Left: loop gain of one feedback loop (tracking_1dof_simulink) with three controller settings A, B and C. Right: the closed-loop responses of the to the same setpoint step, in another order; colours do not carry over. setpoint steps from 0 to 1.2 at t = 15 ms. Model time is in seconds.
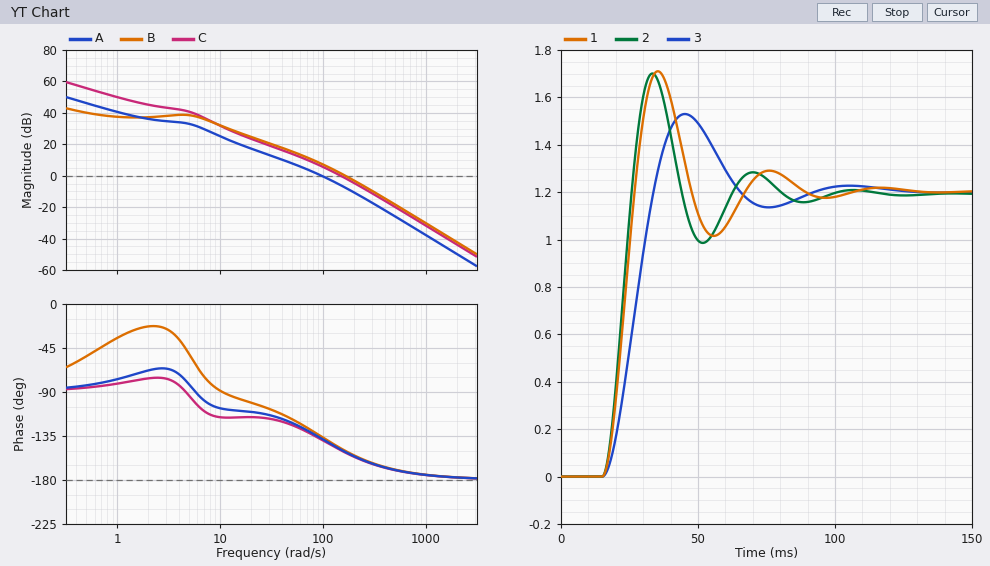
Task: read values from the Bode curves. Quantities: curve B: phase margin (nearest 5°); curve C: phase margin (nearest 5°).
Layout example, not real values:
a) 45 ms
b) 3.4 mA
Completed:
a) 30°
b) 30°
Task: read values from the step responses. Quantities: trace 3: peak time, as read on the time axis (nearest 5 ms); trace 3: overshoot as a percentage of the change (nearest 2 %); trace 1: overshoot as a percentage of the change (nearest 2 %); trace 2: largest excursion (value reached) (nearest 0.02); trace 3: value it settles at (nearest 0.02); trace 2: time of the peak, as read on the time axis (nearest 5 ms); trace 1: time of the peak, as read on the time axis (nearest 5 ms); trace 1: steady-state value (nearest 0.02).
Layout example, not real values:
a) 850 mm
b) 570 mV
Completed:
a) 45 ms
b) 28 %
c) 42 %
d) 1.70
e) 1.20
f) 35 ms
g) 35 ms
h) 1.20
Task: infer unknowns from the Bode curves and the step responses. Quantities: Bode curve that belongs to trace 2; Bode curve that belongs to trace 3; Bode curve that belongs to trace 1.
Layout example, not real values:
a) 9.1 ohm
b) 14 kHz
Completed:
a) B
b) A
c) C
